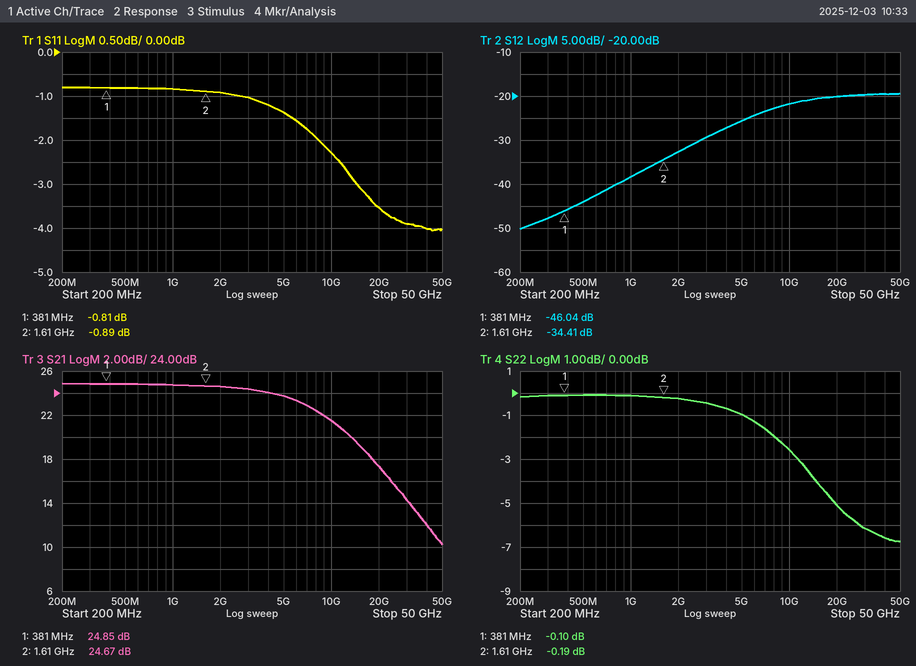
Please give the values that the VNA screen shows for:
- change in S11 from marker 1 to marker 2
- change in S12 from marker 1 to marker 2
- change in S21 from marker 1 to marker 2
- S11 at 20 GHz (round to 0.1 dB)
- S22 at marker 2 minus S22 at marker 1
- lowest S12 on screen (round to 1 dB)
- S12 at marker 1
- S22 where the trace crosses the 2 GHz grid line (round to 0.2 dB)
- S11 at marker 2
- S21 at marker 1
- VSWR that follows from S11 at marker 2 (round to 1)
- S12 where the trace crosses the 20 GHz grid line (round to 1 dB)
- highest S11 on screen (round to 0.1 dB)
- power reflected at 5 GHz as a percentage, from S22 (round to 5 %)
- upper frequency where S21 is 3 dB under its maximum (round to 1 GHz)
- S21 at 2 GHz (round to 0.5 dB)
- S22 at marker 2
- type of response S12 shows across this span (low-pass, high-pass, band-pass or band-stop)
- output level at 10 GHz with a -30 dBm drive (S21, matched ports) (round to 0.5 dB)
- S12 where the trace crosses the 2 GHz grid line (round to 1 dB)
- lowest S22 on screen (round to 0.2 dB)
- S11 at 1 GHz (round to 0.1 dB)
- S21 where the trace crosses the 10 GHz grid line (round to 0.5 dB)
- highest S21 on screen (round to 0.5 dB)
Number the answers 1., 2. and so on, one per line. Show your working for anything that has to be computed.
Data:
1. -0.89 − (-0.81) = -0.08 dB
2. -34.41 − (-46.04) = 11.63 dB
3. 24.67 − (24.85) = -0.18 dB
4. -3.5 dB
5. -0.19 − (-0.1) = -0.09 dB
6. -50 dB
7. -46.04 dB
8. -0.2 dB
9. -0.89 dB
10. 24.85 dB
11. (1 + 0.9026)/(1 − 0.9026) ≈ 20
12. -20 dB
13. -0.8 dB
14. 10^(-1/10) ≈ 79.4 %, so 80 % to the nearest 5 %
15. 9 GHz
16. 24.5 dB
17. -0.19 dB
18. high-pass
19. -30 dBm + (21.5 dB) = -8.5 dBm
20. -33 dB
21. -6.8 dB
22. -0.8 dB
23. 21.5 dB
24. 25.0 dB
